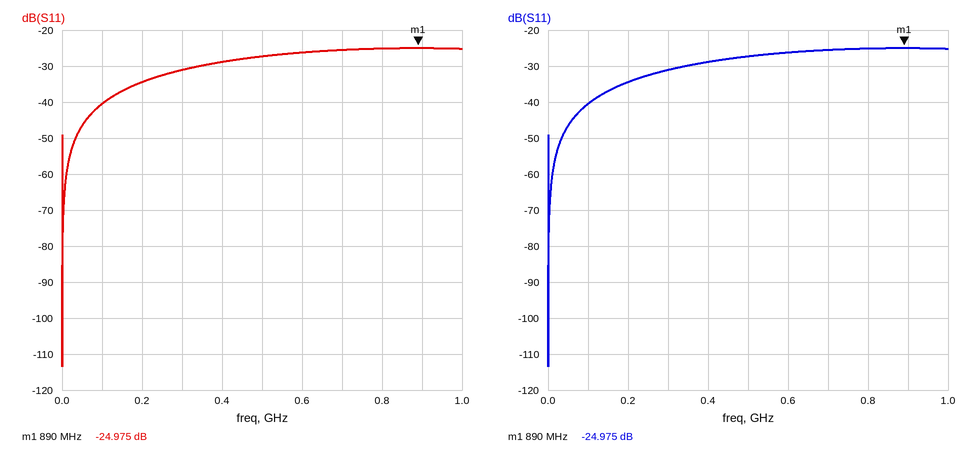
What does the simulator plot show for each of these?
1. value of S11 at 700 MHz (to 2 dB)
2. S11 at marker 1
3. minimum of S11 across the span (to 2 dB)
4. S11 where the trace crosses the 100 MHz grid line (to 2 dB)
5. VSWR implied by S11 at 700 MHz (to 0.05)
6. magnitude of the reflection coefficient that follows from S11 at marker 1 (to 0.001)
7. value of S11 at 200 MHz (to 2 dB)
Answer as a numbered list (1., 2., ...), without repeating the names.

1. -26 dB
2. -24.975 dB
3. -114 dB
4. -40 dB
5. 1.10
6. 0.056
7. -34 dB
